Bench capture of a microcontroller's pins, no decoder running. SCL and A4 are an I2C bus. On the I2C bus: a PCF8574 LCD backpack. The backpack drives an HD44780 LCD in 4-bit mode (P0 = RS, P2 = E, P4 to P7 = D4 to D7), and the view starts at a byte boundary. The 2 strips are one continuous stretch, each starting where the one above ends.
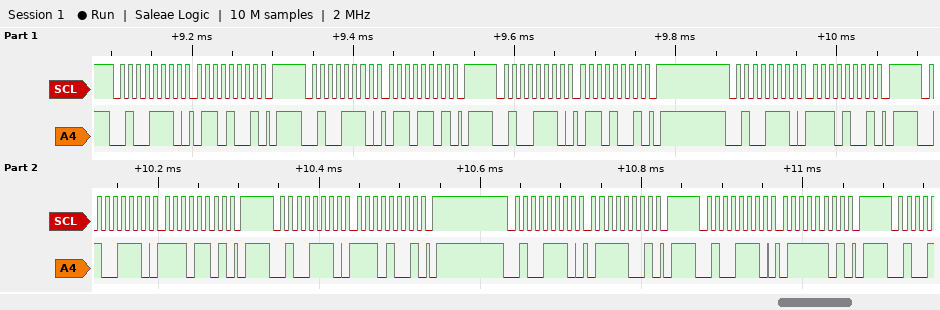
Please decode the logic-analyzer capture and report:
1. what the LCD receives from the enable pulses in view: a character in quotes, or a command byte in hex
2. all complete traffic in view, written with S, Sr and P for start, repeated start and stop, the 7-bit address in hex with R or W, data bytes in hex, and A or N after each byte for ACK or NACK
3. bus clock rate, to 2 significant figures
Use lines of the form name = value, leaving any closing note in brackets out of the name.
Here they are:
what the LCD receives from the enable pulses in view: a character in quotes, or a command byte in hex = 'n'
all complete traffic in view, written with S, Sr and P for start, repeated start and stop, the 7-bit address in hex with R or W, data bytes in hex, and A or N after each byte for ACK or NACK = S 27W A 69 A P S 27W A 6D A P S 27W A 69 A P S 27W A E9 A P S 27W A ED A P S 27W A E9 A P S 27W A 79 A P S 27W A 7D A P
bus clock rate, to 2 significant figures = 100 kHz
